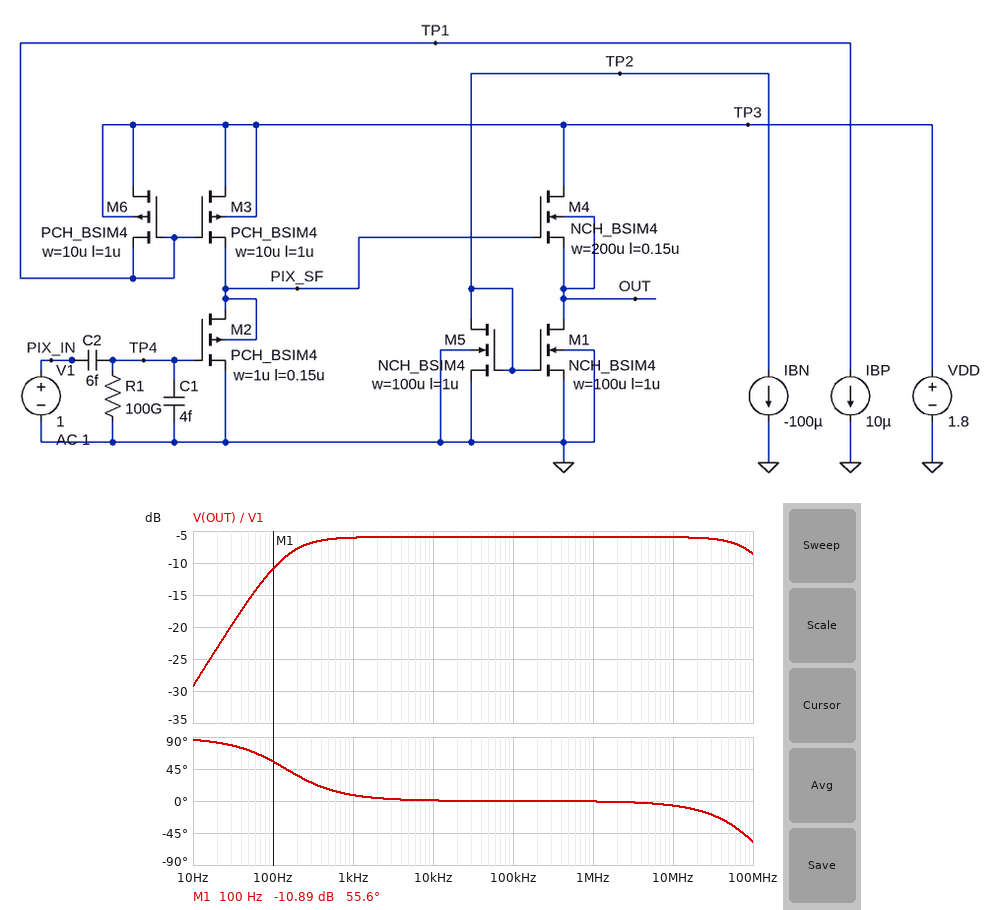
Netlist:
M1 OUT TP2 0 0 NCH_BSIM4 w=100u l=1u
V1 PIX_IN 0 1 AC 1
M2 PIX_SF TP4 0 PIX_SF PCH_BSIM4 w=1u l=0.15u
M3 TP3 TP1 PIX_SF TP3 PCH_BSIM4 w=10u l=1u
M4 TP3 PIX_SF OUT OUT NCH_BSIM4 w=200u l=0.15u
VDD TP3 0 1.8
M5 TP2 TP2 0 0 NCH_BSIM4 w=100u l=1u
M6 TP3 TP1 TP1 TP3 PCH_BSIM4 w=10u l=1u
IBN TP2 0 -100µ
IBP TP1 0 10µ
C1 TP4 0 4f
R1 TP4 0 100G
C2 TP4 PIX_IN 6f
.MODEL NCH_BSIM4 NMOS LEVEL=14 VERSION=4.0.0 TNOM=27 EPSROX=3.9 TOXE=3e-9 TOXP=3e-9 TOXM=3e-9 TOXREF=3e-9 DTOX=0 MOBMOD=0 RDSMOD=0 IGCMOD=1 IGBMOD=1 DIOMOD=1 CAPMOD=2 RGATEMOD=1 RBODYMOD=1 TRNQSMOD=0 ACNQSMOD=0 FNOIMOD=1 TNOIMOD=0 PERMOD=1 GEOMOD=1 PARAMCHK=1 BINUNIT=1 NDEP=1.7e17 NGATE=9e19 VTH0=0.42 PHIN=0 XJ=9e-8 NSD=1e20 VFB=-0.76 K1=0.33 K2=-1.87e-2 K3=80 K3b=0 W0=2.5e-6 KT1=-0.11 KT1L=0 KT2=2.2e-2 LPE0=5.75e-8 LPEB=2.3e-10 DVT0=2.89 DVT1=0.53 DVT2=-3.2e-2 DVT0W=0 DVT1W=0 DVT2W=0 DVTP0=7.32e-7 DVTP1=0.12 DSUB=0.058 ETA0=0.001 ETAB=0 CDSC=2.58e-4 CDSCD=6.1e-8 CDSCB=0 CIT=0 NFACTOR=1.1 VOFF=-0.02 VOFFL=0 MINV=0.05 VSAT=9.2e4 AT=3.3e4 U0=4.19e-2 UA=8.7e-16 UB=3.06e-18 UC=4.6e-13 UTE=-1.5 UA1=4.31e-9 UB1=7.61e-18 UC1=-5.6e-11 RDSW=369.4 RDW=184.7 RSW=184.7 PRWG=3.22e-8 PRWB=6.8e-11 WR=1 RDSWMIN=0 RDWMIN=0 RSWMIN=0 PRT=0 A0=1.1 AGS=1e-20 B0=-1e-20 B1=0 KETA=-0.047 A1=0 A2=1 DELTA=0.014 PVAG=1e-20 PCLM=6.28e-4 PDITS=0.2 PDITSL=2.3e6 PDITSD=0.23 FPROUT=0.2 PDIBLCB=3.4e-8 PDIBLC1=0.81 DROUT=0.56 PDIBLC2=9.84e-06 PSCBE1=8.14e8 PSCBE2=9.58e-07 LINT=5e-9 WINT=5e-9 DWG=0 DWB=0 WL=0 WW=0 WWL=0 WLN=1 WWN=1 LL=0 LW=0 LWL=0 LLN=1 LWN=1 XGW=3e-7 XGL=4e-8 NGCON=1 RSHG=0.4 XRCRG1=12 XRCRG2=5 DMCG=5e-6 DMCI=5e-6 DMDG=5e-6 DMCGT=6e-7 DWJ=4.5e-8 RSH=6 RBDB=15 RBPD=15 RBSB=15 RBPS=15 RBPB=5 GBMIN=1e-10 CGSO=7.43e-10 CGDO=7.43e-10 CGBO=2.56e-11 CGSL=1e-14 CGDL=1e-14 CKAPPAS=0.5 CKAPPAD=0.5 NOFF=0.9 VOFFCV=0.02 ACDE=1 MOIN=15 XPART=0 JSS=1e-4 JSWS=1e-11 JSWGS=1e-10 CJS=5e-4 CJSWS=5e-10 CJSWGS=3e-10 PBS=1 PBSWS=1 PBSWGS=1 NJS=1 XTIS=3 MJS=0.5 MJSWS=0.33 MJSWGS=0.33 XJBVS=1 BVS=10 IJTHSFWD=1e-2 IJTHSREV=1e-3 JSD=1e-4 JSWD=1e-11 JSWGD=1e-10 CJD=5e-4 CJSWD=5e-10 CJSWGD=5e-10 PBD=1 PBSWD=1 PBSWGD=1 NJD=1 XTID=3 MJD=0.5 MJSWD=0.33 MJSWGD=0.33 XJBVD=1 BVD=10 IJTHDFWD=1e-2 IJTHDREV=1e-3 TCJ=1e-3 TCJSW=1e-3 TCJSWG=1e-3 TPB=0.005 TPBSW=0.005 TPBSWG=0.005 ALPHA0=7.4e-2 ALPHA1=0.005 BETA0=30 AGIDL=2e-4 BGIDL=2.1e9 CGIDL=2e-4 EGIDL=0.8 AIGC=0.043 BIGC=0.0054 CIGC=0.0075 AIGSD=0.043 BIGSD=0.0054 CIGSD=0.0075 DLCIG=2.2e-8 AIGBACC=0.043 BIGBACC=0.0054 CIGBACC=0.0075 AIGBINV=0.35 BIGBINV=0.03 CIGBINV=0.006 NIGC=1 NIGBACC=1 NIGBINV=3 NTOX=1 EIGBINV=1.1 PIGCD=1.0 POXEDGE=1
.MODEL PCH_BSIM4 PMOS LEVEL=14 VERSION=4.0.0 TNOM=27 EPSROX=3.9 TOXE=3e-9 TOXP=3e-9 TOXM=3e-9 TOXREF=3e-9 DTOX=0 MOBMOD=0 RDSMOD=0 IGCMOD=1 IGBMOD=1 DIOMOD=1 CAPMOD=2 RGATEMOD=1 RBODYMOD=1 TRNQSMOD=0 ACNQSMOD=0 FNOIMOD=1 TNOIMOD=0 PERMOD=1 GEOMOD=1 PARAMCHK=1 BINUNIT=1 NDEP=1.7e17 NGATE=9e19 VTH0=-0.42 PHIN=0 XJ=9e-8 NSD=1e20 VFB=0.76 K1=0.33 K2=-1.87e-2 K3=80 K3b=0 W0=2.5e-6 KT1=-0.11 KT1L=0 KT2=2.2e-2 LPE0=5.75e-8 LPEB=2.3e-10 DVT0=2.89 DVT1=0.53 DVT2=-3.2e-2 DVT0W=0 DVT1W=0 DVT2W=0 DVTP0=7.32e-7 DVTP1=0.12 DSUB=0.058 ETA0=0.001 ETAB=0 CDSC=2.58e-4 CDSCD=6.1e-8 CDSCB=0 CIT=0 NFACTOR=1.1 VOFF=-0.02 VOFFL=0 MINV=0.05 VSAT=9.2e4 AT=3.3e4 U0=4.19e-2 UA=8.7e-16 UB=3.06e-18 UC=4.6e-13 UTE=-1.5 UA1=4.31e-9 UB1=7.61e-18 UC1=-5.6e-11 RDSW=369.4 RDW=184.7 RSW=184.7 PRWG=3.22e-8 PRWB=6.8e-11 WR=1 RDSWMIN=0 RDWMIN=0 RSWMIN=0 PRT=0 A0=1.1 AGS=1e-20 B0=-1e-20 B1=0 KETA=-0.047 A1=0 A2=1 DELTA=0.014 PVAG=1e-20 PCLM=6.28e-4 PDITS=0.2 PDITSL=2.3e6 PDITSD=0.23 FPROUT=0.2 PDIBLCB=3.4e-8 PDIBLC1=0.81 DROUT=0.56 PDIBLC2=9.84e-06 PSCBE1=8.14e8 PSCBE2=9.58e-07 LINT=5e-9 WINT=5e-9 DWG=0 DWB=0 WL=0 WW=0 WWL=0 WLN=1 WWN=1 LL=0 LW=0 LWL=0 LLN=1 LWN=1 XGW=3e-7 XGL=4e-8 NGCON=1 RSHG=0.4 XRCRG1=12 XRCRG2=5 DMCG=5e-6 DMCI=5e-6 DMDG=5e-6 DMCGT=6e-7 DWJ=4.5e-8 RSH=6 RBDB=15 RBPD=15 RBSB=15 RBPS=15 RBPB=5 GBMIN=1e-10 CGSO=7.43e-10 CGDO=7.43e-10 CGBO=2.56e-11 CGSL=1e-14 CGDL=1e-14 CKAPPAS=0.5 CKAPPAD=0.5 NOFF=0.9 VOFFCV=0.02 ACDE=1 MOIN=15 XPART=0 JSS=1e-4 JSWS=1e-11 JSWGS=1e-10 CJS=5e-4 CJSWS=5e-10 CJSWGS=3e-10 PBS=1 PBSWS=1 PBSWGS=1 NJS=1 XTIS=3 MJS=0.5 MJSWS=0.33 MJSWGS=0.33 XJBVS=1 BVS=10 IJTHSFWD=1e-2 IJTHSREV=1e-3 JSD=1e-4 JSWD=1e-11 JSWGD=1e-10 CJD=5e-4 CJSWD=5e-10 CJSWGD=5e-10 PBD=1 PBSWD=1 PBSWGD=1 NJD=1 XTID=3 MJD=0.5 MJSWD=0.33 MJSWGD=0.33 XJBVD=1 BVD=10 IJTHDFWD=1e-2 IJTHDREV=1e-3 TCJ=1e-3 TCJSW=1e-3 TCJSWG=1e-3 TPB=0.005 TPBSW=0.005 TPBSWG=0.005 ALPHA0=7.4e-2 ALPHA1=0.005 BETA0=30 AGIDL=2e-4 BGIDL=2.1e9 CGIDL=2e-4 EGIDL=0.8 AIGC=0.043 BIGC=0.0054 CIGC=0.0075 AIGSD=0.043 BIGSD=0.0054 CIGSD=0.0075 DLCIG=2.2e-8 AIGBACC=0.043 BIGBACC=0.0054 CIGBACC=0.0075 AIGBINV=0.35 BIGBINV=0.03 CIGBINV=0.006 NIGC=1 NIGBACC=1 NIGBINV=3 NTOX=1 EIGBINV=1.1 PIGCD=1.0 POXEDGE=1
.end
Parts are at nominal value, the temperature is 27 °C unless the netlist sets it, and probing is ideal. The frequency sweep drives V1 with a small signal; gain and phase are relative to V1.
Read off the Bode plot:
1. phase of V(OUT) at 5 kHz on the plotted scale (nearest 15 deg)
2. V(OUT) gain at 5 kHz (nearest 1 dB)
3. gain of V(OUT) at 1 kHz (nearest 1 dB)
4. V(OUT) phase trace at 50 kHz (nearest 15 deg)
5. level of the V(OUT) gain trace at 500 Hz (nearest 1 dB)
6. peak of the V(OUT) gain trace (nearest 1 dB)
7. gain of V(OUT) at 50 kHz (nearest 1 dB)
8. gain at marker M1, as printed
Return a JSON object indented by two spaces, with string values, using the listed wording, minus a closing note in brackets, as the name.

{
  "phase of V(OUT) at 5 kHz on the plotted scale": "0 deg",
  "V(OUT) gain at 5 kHz": "-6 dB",
  "gain of V(OUT) at 1 kHz": "-6 dB",
  "V(OUT) phase trace at 50 kHz": "0 deg",
  "level of the V(OUT) gain trace at 500 Hz": "-6 dB",
  "peak of the V(OUT) gain trace": "-6 dB",
  "gain of V(OUT) at 50 kHz": "-6 dB",
  "gain at marker M1, as printed": "-10.89 dB"
}
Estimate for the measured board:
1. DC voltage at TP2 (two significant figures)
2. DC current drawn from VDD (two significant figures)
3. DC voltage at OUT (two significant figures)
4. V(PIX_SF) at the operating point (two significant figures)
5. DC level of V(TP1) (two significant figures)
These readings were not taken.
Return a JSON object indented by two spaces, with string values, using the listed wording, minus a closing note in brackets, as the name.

{
  "DC voltage at TP2": "590 mV",
  "DC current drawn from VDD": "120 µA",
  "DC voltage at OUT": "220 mV",
  "V(PIX_SF) at the operating point": "690 mV",
  "DC level of V(TP1)": "1.2 V"
}
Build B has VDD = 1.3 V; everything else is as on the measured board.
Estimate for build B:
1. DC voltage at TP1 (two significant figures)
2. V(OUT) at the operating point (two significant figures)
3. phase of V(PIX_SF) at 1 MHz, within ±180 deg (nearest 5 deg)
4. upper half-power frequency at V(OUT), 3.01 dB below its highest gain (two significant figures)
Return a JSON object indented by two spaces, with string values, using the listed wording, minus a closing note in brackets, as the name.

{
  "DC voltage at TP1": "700 mV",
  "V(OUT) at the operating point": "200 mV",
  "phase of V(PIX_SF) at 1 MHz, within ±180 deg": "0 deg",
  "upper half-power frequency at V(OUT), 3.01 dB below its highest gain": "100 MHz"
}
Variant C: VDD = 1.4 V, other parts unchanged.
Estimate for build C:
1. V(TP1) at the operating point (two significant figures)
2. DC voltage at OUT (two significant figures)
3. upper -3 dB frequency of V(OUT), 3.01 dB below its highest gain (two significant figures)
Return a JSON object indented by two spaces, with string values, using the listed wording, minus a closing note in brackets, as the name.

{
  "V(TP1) at the operating point": "800 mV",
  "DC voltage at OUT": "200 mV",
  "upper -3 dB frequency of V(OUT), 3.01 dB below its highest gain": "100 MHz"
}
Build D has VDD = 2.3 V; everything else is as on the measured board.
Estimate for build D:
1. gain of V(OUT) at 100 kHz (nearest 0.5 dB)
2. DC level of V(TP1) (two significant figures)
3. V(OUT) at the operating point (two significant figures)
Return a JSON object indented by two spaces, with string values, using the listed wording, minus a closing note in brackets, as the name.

{
  "gain of V(OUT) at 100 kHz": "-6.5 dB",
  "DC level of V(TP1)": "1.7 V",
  "V(OUT) at the operating point": "240 mV"
}
